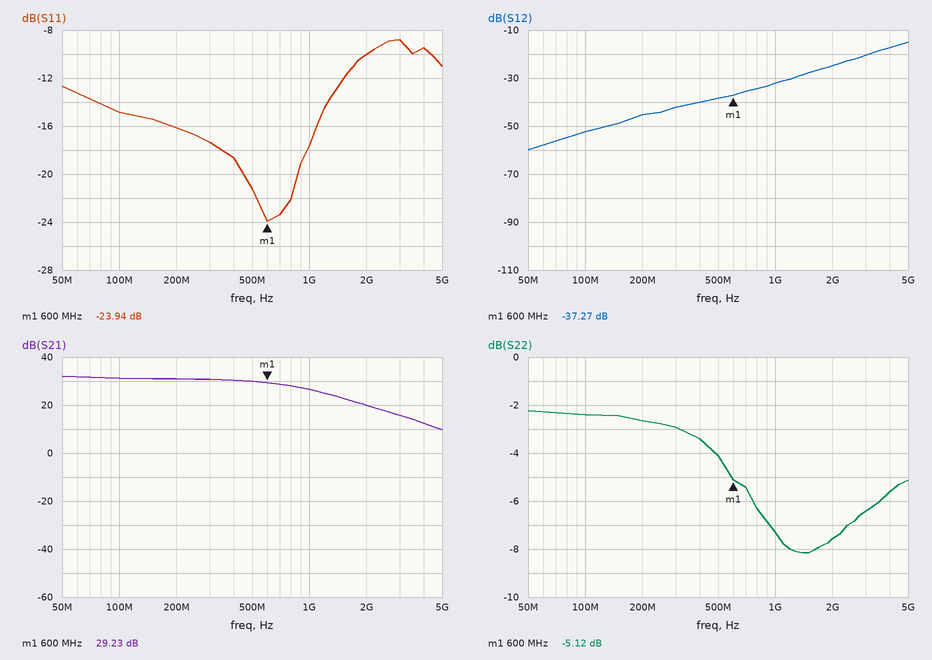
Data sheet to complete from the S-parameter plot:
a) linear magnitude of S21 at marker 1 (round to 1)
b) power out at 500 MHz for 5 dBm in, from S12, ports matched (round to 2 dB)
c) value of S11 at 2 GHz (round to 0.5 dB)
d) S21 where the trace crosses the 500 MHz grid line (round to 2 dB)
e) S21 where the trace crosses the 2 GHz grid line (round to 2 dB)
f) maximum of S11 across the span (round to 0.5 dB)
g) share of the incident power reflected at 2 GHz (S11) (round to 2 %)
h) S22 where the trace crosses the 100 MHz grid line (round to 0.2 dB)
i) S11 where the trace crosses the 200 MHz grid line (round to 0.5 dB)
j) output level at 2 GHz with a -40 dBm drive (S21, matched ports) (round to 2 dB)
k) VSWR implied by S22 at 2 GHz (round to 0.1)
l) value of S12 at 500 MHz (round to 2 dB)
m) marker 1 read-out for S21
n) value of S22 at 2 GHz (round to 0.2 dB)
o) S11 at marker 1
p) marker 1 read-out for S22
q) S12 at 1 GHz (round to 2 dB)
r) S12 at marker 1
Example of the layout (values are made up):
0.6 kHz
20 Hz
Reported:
29
-34 dBm
-10.0 dB
30 dB
20 dB
-9.0 dB
10 %
-2.4 dB
-16.0 dB
-20 dBm
2.4
-38 dB
29.23 dB
-7.6 dB
-23.94 dB
-5.12 dB
-32 dB
-37.27 dB
